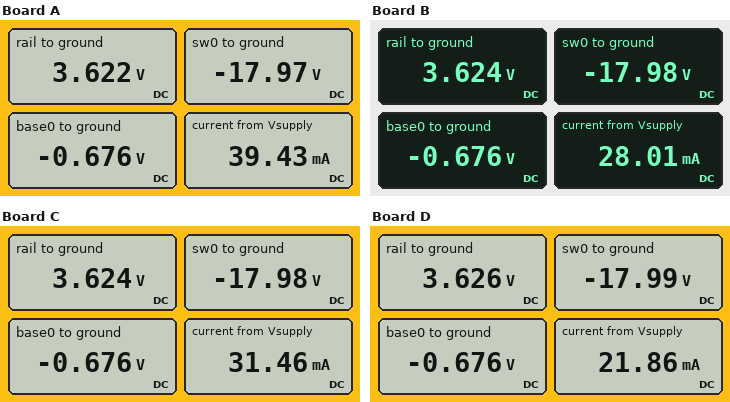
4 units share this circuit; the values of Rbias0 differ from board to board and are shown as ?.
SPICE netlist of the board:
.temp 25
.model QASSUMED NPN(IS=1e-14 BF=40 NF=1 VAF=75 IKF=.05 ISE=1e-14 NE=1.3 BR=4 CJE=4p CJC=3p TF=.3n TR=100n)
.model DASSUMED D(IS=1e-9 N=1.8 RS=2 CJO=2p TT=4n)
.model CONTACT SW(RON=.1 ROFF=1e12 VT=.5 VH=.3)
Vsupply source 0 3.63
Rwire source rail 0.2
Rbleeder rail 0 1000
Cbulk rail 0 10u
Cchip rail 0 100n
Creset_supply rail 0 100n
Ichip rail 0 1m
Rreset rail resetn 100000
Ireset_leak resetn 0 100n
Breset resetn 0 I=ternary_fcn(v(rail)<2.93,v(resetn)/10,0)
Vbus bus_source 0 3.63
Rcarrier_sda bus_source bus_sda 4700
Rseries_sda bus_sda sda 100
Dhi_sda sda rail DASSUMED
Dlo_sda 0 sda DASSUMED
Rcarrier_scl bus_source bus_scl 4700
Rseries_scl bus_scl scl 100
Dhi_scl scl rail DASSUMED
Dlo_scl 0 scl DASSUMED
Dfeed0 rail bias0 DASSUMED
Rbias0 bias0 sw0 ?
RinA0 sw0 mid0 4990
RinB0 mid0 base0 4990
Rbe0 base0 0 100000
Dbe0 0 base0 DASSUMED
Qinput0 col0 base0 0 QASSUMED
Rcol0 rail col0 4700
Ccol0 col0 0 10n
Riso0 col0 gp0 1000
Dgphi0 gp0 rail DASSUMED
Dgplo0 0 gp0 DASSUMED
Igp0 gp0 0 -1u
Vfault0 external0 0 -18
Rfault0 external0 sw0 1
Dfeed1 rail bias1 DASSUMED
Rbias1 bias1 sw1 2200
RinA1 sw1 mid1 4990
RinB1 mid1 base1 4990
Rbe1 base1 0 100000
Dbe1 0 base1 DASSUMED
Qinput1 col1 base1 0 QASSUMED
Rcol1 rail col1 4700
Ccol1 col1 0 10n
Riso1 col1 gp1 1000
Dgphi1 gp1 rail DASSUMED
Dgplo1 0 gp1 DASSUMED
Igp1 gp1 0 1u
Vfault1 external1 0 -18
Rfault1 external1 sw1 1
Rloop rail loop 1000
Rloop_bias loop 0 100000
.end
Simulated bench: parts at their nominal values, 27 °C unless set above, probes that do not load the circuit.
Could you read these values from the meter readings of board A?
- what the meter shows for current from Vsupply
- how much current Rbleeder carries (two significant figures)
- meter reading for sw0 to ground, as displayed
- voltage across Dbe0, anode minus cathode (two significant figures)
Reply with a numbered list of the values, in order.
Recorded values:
1. 39.43 mA
2. 3.6 mA
3. -17.97 V
4. 680 mV
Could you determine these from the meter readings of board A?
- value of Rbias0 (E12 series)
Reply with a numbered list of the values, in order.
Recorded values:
1. 820 Ω
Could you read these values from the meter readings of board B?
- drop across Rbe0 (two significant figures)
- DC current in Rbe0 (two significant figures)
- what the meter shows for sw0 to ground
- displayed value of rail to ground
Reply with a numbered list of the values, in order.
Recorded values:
1. 680 mV
2. 6.8 µA
3. -17.98 V
4. 3.624 V
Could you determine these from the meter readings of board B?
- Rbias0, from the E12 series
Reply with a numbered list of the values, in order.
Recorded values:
1. 1.5 kΩ
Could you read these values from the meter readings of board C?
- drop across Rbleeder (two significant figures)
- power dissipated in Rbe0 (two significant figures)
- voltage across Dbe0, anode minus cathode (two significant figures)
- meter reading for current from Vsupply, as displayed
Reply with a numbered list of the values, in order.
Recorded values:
1. 3.6 V
2. 4.6 µW
3. 680 mV
4. 31.46 mA
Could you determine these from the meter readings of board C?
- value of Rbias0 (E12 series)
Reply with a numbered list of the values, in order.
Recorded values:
1. 1.2 kΩ
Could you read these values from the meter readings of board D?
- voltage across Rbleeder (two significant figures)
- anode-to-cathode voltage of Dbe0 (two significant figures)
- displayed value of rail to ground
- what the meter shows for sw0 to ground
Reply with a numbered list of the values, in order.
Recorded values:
1. 3.6 V
2. 680 mV
3. 3.626 V
4. -17.99 V
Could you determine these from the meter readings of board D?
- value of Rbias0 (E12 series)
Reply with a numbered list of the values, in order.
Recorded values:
1. 2.7 kΩ
